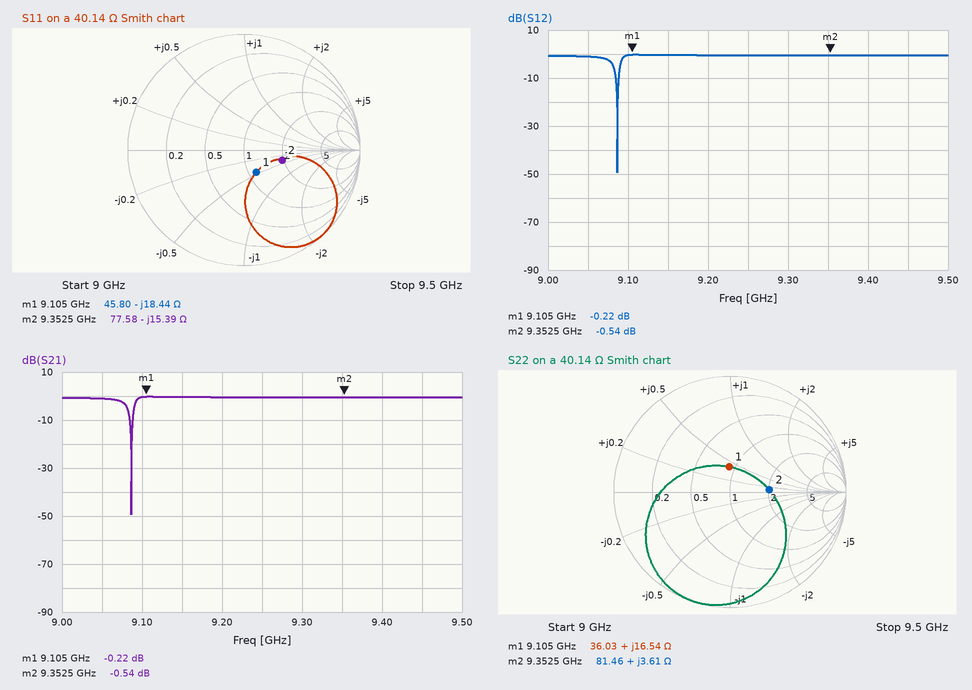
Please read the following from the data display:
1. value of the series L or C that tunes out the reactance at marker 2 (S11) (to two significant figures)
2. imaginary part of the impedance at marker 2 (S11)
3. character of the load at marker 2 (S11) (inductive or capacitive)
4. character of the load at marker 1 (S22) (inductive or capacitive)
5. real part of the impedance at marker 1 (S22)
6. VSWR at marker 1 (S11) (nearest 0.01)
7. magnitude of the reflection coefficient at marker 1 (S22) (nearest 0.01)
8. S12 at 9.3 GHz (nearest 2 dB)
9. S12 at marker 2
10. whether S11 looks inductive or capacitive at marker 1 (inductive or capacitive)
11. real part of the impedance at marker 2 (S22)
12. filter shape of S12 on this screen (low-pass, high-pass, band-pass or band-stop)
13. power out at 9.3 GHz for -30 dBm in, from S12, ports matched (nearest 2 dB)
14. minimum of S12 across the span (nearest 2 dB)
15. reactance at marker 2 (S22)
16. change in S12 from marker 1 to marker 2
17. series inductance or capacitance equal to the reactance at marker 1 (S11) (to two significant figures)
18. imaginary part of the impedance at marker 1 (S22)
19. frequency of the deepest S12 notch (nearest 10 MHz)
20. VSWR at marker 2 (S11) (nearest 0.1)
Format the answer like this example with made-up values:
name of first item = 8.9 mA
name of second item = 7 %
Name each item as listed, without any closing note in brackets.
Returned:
value of the series L or C that tunes out the reactance at marker 2 (S11) = 260 pH
imaginary part of the impedance at marker 2 = -15.39 Ω
character of the load at marker 2 (S11) = capacitive
character of the load at marker 1 (S22) = inductive
real part of the impedance at marker 1 = 36.03 Ω
VSWR at marker 1 (S11) = 1.56
magnitude of the reflection coefficient at marker 1 (S22) = 0.22
S12 at 9.3 GHz = 0 dB
S12 at marker 2 = -0.54 dB
whether S11 looks inductive or capacitive at marker 1 = capacitive
real part of the impedance at marker 2 = 81.46 Ω
filter shape of S12 on this screen = band-stop
power out at 9.3 GHz for -30 dBm in, from S12, ports matched = -30 dBm
minimum of S12 across the span = -50 dB
reactance at marker 2 = +3.61 Ω
change in S12 from marker 1 to marker 2 = -0.32 dB
series inductance or capacitance equal to the reactance at marker 1 (S11) = 950 fF
imaginary part of the impedance at marker 1 = +16.54 Ω
frequency of the deepest S12 notch = 9.09 GHz
VSWR at marker 2 (S11) = 2.0
